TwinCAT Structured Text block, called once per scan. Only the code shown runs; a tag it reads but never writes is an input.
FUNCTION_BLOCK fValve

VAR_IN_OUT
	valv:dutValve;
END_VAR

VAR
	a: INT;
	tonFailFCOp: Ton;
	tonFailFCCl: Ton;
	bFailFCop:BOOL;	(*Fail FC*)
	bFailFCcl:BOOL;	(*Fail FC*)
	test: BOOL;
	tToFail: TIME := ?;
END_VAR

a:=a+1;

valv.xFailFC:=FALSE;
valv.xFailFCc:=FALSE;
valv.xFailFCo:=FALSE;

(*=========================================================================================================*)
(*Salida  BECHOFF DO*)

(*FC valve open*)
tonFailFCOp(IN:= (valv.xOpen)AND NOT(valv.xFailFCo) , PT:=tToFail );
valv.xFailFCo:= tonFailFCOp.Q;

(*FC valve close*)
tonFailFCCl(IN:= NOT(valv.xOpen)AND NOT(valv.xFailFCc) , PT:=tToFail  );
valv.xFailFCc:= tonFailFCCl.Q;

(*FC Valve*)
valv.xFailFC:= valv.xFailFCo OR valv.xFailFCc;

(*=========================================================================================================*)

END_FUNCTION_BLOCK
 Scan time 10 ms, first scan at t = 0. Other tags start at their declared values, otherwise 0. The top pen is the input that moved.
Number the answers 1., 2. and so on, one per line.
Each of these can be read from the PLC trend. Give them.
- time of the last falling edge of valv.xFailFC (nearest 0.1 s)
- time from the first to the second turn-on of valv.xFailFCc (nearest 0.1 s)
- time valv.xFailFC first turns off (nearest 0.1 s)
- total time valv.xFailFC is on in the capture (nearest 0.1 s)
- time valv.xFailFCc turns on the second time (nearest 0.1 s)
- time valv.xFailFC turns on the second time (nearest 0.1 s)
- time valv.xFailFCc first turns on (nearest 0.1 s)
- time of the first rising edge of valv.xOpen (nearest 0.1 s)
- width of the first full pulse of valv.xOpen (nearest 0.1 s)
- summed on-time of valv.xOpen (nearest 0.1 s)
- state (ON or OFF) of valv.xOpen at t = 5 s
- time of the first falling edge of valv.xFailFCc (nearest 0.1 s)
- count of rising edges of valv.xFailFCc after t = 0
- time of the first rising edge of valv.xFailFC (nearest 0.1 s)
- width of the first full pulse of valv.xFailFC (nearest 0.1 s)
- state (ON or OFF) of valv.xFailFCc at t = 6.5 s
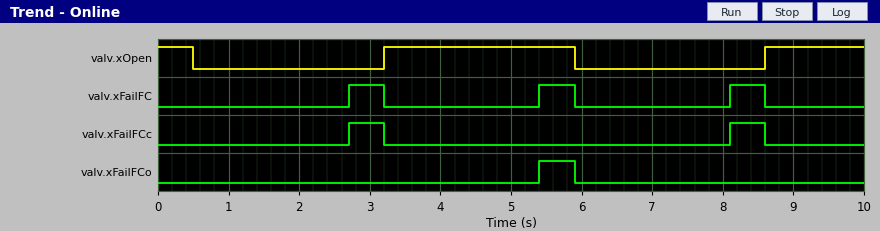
1. 8.6 s
2. 5.4 s
3. 3.2 s
4. 1.5 s
5. 8.1 s
6. 5.4 s
7. 2.7 s
8. 3.2 s
9. 2.7 s
10. 4.6 s
11. ON
12. 3.2 s
13. 2
14. 2.7 s
15. 0.5 s
16. OFF
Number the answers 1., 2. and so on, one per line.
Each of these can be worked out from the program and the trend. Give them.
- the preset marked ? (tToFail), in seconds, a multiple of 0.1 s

1. 2.2 s
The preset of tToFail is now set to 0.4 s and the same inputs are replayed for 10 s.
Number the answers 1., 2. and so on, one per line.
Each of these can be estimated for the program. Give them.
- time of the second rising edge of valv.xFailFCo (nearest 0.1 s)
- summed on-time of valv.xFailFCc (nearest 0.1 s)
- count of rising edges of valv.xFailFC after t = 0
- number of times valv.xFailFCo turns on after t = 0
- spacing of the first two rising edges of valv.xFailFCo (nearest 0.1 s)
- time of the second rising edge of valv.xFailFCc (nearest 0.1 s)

1. 3.6 s
2. 4.6 s
3. 5
4. 3
5. 3.2 s
6. 6.3 s
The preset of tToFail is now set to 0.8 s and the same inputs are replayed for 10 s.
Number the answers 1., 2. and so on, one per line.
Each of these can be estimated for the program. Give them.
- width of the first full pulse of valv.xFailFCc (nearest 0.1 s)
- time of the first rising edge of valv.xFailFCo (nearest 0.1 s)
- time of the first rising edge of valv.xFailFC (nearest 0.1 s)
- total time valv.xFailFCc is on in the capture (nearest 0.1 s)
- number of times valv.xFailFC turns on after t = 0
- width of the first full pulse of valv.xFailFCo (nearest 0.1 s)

1. 1.9 s
2. 4.0 s
3. 1.3 s
4. 3.8 s
5. 4
6. 1.9 s
